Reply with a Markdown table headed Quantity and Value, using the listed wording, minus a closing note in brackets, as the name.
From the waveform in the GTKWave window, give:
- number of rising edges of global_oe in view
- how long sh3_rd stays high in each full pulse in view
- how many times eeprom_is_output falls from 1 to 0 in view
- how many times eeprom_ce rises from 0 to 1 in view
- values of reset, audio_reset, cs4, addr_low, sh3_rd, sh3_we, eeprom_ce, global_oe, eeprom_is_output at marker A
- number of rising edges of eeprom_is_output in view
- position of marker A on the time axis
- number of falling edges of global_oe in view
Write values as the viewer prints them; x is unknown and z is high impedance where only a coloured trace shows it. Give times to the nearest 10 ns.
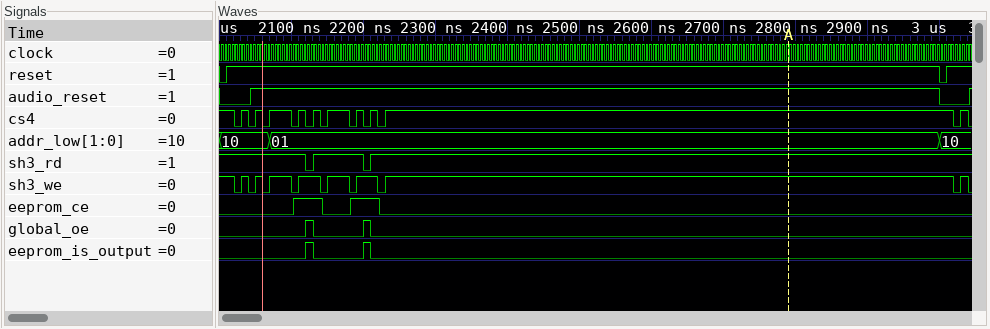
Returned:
| Quantity | Value |
|---|---|
| number of rising edges of global_oe in view | 2 |
| how long sh3_rd stays high in each full pulse in view | 70 ns |
| how many times eeprom_is_output falls from 1 to 0 in view | 2 |
| how many times eeprom_ce rises from 0 to 1 in view | 2 |
| values of reset, audio_reset, cs4, addr_low, sh3_rd, sh3_we, eeprom_ce, global_oe, eeprom_is_output at marker A | reset=1, audio_reset=1, cs4=1, addr_low=01, sh3_rd=1, sh3_we=1, eeprom_ce=0, global_oe=0, eeprom_is_output=0 |
| number of rising edges of eeprom_is_output in view | 2 |
| position of marker A on the time axis | 2790 ns |
| number of falling edges of global_oe in view | 2 |
